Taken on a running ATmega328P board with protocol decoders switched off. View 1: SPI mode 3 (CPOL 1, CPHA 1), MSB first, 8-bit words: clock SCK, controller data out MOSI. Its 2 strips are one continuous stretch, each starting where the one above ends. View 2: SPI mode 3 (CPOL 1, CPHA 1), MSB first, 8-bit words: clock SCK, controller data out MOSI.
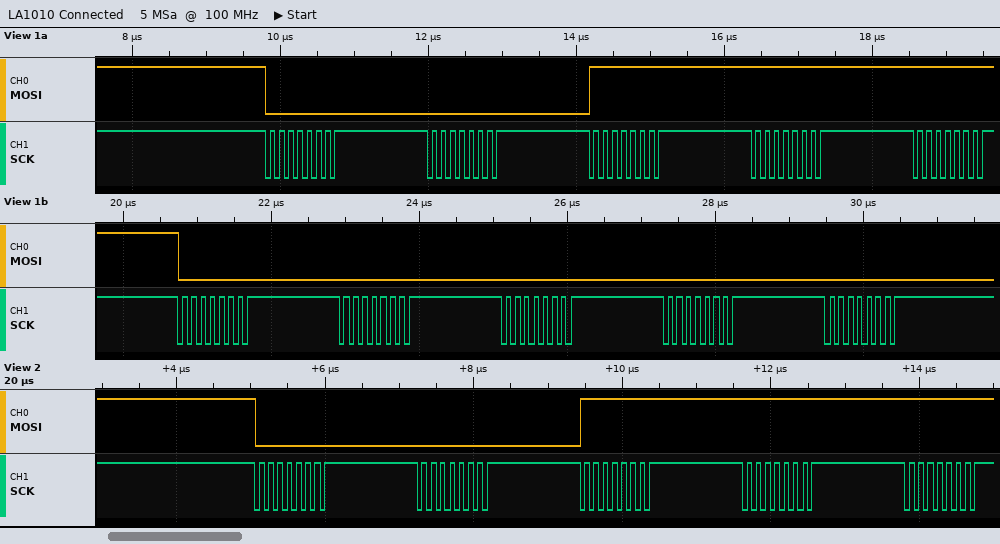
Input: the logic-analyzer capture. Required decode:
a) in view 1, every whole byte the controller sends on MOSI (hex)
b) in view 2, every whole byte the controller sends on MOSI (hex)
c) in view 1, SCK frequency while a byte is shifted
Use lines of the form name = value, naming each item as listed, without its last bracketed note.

in view 1, every whole byte the controller sends on MOSI = 00 00 FF FF FF 00 00 00 00 00
in view 2, every whole byte the controller sends on MOSI = 00 00 FF FF FF
in view 1, SCK frequency while a byte is shifted = 8 MHz
